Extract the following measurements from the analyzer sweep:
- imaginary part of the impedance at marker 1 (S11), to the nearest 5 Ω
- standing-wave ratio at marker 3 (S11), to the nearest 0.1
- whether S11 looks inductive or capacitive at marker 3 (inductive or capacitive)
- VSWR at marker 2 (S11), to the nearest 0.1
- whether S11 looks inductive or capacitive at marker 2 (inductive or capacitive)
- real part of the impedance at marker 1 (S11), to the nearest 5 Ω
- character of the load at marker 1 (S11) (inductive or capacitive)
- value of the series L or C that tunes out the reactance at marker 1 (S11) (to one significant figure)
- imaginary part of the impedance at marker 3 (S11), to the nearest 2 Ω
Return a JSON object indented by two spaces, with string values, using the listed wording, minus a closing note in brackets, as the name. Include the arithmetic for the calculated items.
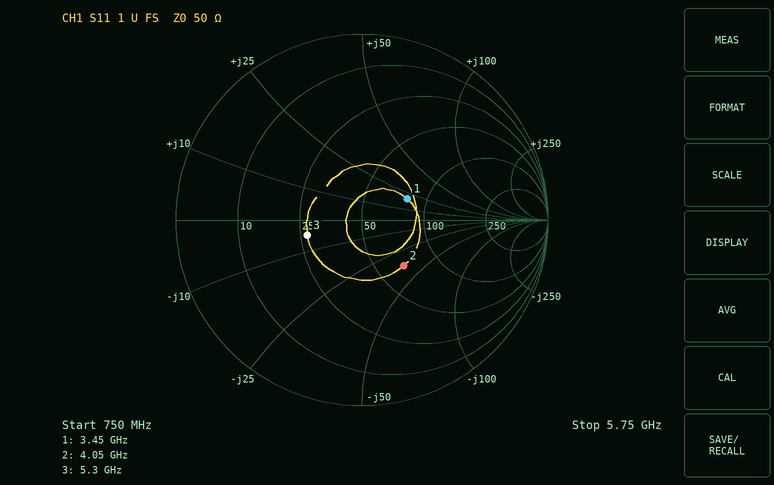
{
  "imaginary part of the impedance at marker 1 (S11), to the nearest 5 Ω": "+20 Ω",
  "standing-wave ratio at marker 3 (S11), to the nearest 0.1": "1.9",
  "whether S11 looks inductive or capacitive at marker 3": "capacitive",
  "VSWR at marker 2 (S11), to the nearest 0.1": "2.0",
  "whether S11 looks inductive or capacitive at marker 2": "capacitive",
  "real part of the impedance at marker 1 (S11), to the nearest 5 Ω": "80 Ω",
  "character of the load at marker 1 (S11)": "inductive",
  "value of the series L or C that tunes out the reactance at marker 1 (S11)": "C = 1/(2π × 3.45 GHz × 20 Ω) ≈ 2 pF",
  "imaginary part of the impedance at marker 3 (S11), to the nearest 2 Ω": "-4 Ω"
}
